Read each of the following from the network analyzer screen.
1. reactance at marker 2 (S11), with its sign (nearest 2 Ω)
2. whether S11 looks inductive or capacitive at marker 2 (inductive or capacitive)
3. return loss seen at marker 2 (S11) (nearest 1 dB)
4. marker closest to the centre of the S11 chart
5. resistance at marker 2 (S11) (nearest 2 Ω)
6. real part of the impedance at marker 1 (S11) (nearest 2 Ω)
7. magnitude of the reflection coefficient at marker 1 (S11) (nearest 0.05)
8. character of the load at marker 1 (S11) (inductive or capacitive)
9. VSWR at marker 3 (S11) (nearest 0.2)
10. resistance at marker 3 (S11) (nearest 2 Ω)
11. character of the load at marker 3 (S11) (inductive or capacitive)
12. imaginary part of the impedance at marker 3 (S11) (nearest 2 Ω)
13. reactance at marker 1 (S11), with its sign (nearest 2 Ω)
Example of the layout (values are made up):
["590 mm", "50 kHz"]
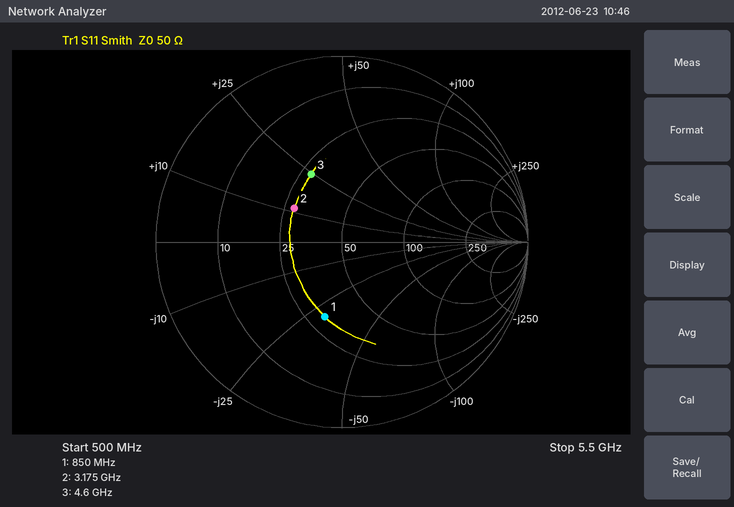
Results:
["+12 Ω", "inductive", "10 dB", "marker 2", "28 Ω", "30 Ω", "0.40", "capacitive", "2.4", "28 Ω", "inductive", "+24 Ω", "-30 Ω"]
